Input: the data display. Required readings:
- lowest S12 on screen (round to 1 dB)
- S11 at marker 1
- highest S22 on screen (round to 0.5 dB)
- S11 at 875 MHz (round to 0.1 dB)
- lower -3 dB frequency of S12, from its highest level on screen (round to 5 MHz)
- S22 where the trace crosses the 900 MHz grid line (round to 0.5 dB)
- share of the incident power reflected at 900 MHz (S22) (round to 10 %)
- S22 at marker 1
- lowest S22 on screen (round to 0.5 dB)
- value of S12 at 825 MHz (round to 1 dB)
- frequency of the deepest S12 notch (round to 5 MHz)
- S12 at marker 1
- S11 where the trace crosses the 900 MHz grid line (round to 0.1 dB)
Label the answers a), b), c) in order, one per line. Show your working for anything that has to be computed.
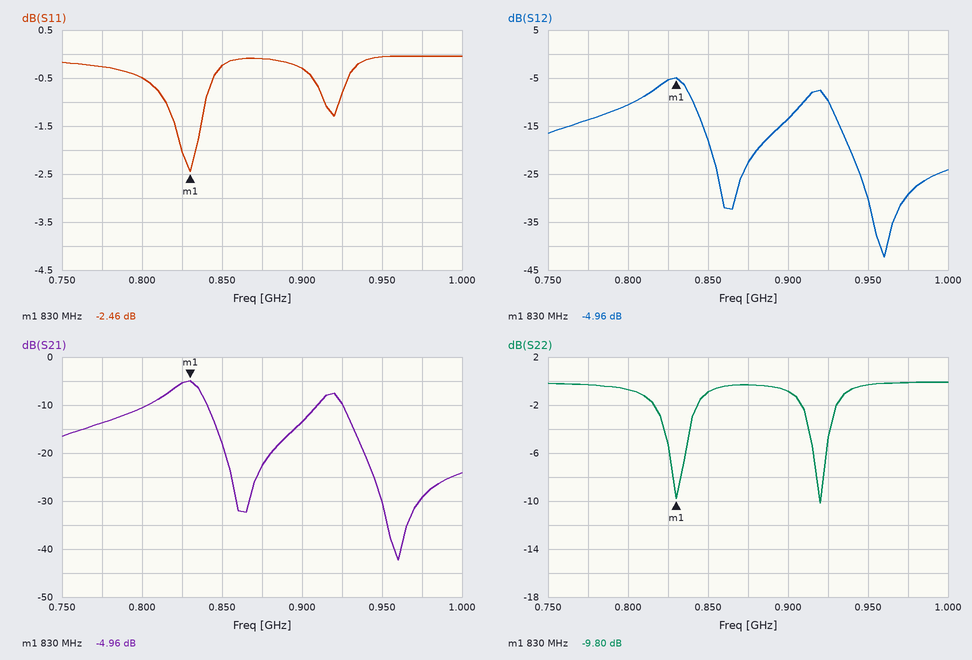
a) -42 dB
b) -2.46 dB
c) 0.0 dB
d) -0.1 dB
e) 815 MHz
f) -1.0 dB
g) 10^(-1/10) ≈ 79.4 %, so 80 % to the nearest 10 %
h) -9.80 dB
i) -10.0 dB
j) -5 dB
k) 960 MHz
l) -4.96 dB
m) -0.3 dB
